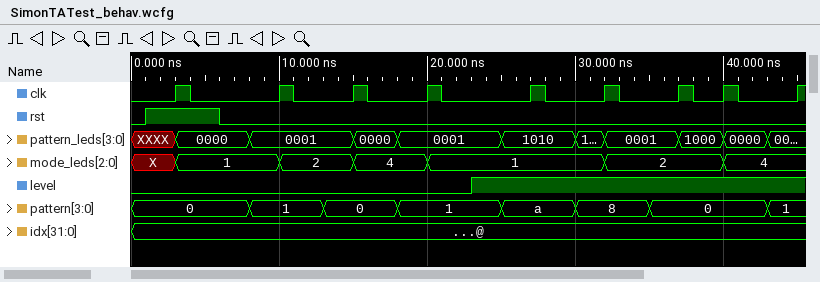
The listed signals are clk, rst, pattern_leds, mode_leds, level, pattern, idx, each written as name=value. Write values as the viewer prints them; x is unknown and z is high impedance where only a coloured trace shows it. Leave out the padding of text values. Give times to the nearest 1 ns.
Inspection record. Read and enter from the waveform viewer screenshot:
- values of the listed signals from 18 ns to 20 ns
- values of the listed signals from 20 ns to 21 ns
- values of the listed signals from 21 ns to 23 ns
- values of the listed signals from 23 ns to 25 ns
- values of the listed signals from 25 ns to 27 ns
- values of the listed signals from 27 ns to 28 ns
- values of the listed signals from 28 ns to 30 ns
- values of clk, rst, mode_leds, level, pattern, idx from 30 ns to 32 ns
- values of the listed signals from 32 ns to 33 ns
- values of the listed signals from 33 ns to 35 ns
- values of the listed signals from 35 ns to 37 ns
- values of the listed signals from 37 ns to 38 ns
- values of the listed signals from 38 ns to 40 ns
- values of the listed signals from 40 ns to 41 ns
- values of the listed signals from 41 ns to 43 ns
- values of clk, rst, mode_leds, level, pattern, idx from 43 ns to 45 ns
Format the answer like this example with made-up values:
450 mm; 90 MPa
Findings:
clk=0, rst=0, pattern_leds=0001, mode_leds=4, level=0, pattern=1, idx=@; clk=1, rst=0, pattern_leds=0001, mode_leds=1, level=0, pattern=1, idx=@; clk=0, rst=0, pattern_leds=0001, mode_leds=1, level=0, pattern=1, idx=@; clk=0, rst=0, pattern_leds=0001, mode_leds=1, level=1, pattern=1, idx=@; clk=0, rst=0, pattern_leds=1010, mode_leds=1, level=1, pattern=a, idx=@; clk=1, rst=0, pattern_leds=1010, mode_leds=1, level=1, pattern=a, idx=@; clk=0, rst=0, pattern_leds=1010, mode_leds=1, level=1, pattern=a, idx=@; clk=0, rst=0, mode_leds=1, level=1, pattern=8, idx=@; clk=1, rst=0, pattern_leds=0001, mode_leds=2, level=1, pattern=8, idx=@; clk=0, rst=0, pattern_leds=0001, mode_leds=2, level=1, pattern=8, idx=@; clk=0, rst=0, pattern_leds=0001, mode_leds=2, level=1, pattern=0, idx=@; clk=1, rst=0, pattern_leds=1000, mode_leds=2, level=1, pattern=0, idx=@; clk=0, rst=0, pattern_leds=1000, mode_leds=2, level=1, pattern=0, idx=@; clk=1, rst=0, pattern_leds=0000, mode_leds=4, level=1, pattern=0, idx=@; clk=0, rst=0, pattern_leds=0000, mode_leds=4, level=1, pattern=0, idx=@; clk=0, rst=0, mode_leds=4, level=1, pattern=1, idx=@
